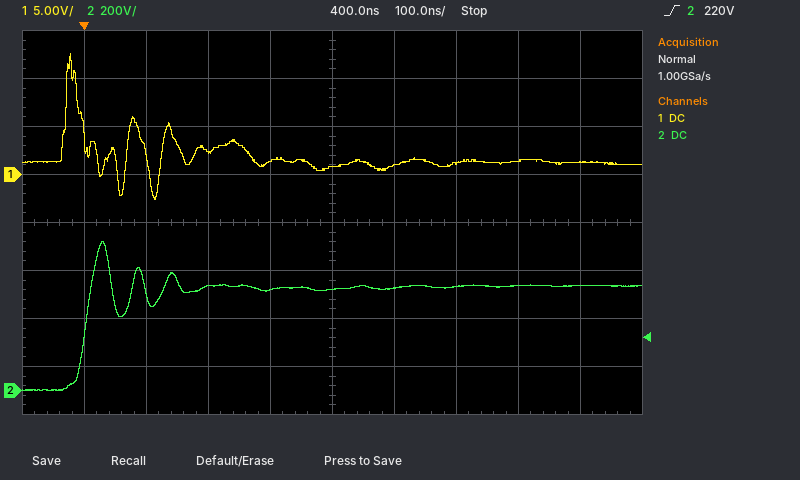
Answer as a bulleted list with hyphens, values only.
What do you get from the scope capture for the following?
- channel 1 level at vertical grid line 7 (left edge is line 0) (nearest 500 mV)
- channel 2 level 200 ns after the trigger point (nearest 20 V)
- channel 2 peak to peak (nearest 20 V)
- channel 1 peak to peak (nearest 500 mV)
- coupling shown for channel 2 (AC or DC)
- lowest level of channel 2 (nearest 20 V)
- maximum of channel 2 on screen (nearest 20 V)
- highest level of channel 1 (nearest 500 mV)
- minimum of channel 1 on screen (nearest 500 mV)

- 1.0 V
- 440 V
- 620 V
- 15.0 V
- DC
- 0 V
- 620 V
- 12.5 V
- -2.5 V
